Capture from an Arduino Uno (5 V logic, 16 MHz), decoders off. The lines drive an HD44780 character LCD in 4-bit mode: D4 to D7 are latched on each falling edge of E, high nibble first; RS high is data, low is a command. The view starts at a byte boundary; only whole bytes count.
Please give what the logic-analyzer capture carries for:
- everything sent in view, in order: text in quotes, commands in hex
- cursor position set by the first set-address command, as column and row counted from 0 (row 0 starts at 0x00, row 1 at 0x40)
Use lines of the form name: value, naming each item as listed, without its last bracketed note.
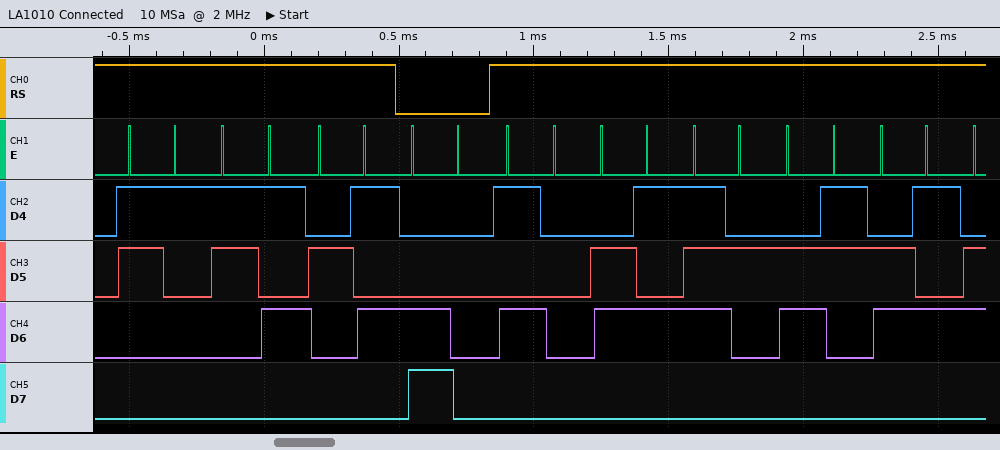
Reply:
everything sent in view, in order: text in quotes, commands in hex: "15%" 0xC0 "Perce"
cursor position set by the first set-address command, as column and row counted from 0: column 0, row 1
